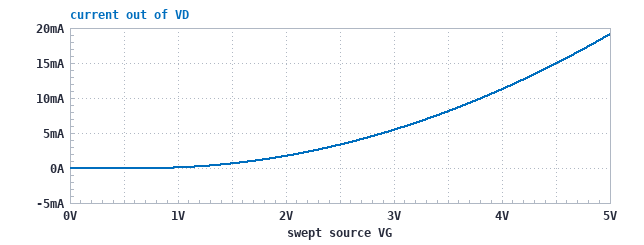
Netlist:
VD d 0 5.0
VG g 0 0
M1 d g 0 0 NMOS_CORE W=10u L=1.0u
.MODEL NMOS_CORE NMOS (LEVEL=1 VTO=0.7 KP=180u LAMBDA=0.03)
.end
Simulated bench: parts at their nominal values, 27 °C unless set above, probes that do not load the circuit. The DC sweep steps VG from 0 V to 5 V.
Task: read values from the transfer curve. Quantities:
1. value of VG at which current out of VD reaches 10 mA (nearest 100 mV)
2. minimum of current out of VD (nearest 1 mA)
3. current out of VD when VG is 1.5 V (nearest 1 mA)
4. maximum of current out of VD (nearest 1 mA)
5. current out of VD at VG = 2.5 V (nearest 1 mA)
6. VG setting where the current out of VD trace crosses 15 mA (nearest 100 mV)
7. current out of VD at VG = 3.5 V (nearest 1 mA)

3.8 V
0 A
1 mA
19 mA
3 mA
4.5 V
8 mA
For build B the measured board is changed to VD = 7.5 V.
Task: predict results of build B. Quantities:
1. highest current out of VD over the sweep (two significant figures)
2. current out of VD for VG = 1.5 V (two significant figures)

20 mA
710 µA
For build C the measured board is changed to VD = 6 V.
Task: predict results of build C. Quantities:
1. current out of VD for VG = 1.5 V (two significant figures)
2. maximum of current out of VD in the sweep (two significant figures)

680 µA
20 mA
